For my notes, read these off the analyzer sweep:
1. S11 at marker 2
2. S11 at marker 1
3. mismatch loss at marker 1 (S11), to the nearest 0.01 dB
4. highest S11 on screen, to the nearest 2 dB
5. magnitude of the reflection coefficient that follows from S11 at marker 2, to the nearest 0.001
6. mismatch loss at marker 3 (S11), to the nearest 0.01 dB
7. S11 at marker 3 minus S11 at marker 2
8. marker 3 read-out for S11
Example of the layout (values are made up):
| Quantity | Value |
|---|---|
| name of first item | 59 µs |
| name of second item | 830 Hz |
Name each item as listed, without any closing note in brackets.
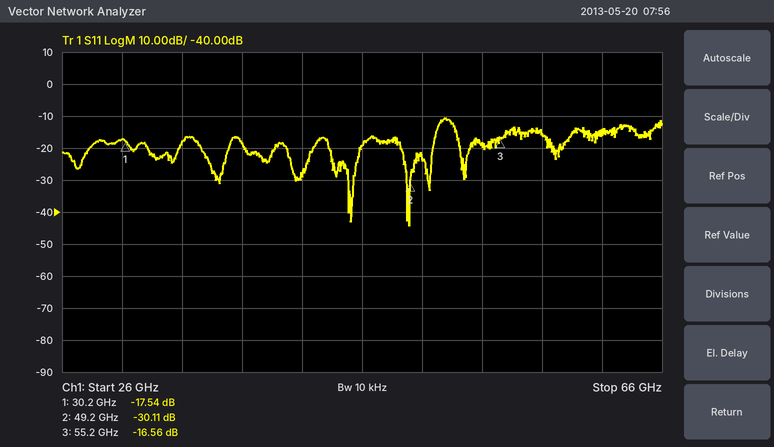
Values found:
| Quantity | Value |
|---|---|
| S11 at marker 2 | -30.11 dB |
| S11 at marker 1 | -17.54 dB |
| mismatch loss at marker 1 (S11), to the nearest 0.01 dB | 0.08 dB |
| highest S11 on screen, to the nearest 2 dB | -10 dB |
| magnitude of the reflection coefficient that follows from S11 at marker 2, to the nearest 0.001 | 0.031 |
| mismatch loss at marker 3 (S11), to the nearest 0.01 dB | 0.10 dB |
| S11 at marker 3 minus S11 at marker 2 | 13.55 dB |
| marker 3 read-out for S11 | -16.56 dB |
